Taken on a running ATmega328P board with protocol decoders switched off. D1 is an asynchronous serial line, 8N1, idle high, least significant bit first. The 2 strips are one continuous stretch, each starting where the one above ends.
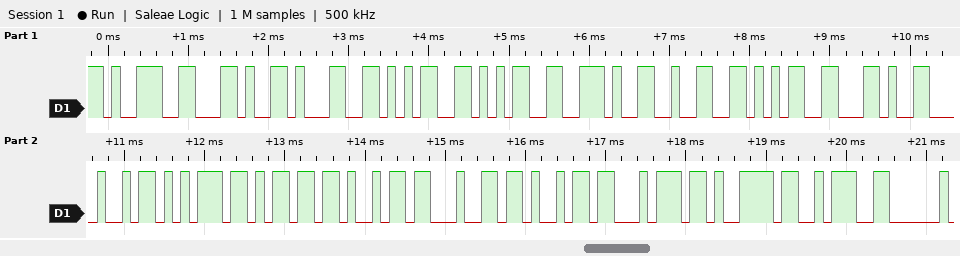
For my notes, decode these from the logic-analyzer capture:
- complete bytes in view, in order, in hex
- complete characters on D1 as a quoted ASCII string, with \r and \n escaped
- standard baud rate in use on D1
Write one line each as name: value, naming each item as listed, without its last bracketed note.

complete bytes in view, in order, in hex: 39 2C 31 35 35 2E 32 35 2C 48 75 6D 69 64 69 74 79 3A
complete characters on D1 as a quoted ASCII string, with \r and \n escaped: "9,155.25,Humidity:"
standard baud rate in use on D1: 9600 baud
